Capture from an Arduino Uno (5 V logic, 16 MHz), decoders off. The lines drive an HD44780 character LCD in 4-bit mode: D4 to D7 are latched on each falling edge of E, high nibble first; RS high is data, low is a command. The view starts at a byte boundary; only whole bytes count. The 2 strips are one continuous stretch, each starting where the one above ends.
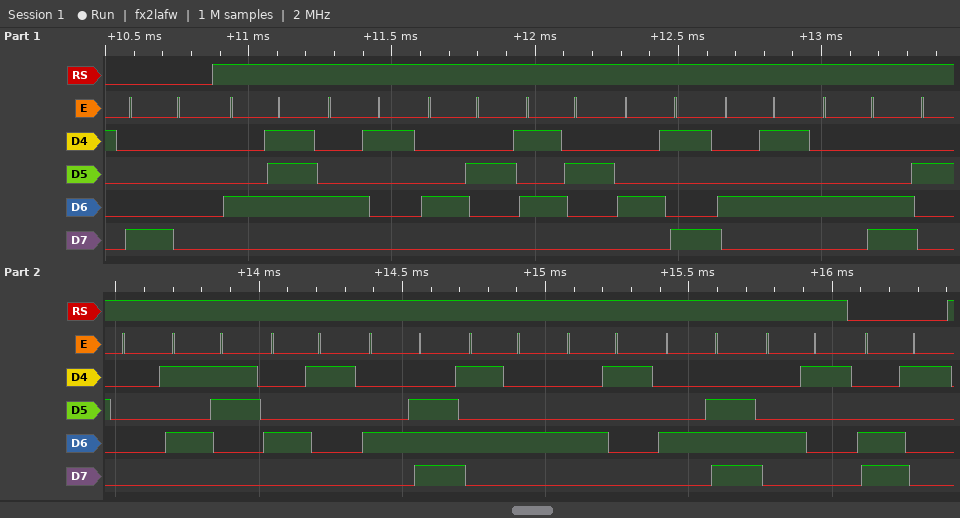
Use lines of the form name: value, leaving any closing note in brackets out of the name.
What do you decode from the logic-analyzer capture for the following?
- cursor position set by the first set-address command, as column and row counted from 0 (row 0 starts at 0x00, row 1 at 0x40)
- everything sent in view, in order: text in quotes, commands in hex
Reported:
cursor position set by the first set-address command, as column and row counted from 0: column 0, row 0
everything sent in view, in order: text in quotes, commands in hex: 0x80 "GABRIEL SANTANA" 0xC1
